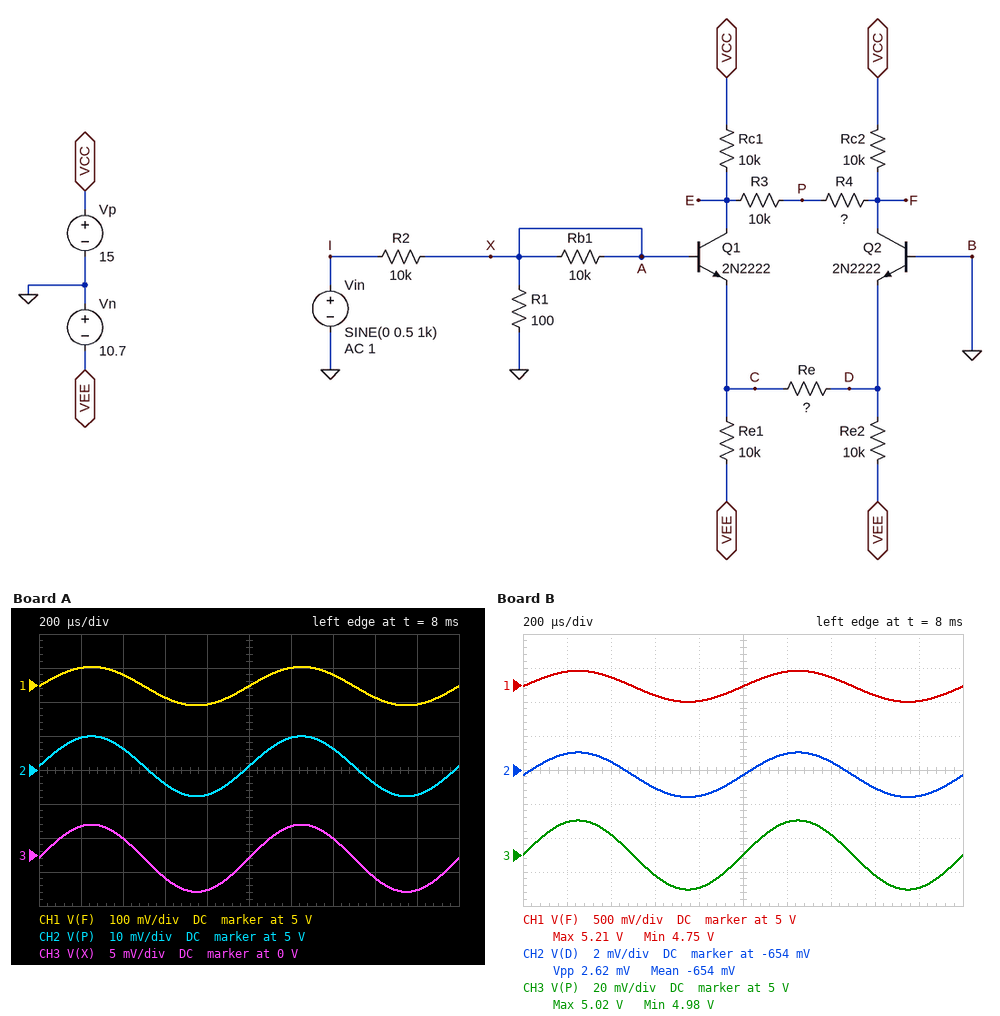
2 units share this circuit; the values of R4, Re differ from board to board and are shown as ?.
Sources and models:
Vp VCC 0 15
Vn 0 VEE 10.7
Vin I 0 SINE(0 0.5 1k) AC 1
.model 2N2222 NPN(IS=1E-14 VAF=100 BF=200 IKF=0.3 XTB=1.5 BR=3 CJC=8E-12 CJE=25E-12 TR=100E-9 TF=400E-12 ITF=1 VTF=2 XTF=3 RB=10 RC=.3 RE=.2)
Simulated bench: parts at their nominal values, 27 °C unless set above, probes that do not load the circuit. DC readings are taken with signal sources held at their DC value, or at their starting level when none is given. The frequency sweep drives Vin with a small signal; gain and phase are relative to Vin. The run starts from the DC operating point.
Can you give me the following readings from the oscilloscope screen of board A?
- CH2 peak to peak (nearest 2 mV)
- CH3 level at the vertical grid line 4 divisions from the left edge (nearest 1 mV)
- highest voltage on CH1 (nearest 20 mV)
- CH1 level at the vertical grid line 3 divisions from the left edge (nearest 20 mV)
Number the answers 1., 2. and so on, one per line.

1. 18 mV
2. -5 mV
3. 5.06 V
4. 4.96 V
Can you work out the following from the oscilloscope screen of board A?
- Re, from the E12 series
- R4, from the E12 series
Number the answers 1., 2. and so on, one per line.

1. 330 Ω
2. 6.8 kΩ
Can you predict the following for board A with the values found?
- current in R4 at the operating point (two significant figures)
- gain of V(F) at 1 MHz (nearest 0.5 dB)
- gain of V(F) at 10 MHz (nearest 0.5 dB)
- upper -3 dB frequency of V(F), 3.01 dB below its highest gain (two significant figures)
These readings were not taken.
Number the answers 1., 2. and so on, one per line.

1. 670 nA
2. -19.0 dB
3. -24.0 dB
4. 6.7 MHz
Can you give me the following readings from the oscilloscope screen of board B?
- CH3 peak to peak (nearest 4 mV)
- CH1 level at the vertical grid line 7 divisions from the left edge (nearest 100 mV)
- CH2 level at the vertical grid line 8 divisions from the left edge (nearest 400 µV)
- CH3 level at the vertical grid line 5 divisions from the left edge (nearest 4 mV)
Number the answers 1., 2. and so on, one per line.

1. 40 mV
2. 5.1 V
3. -655.2 mV
4. 5.000 V
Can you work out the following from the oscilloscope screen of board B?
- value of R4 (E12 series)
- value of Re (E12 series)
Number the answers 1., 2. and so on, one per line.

1. 8.2 kΩ
2. 47 Ω
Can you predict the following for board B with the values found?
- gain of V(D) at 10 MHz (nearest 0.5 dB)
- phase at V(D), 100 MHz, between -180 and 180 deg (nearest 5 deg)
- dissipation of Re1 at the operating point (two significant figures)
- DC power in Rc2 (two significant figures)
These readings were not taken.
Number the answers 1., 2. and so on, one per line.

1. -55.5 dB
2. -20 deg
3. 10 mW
4. 10 mW
